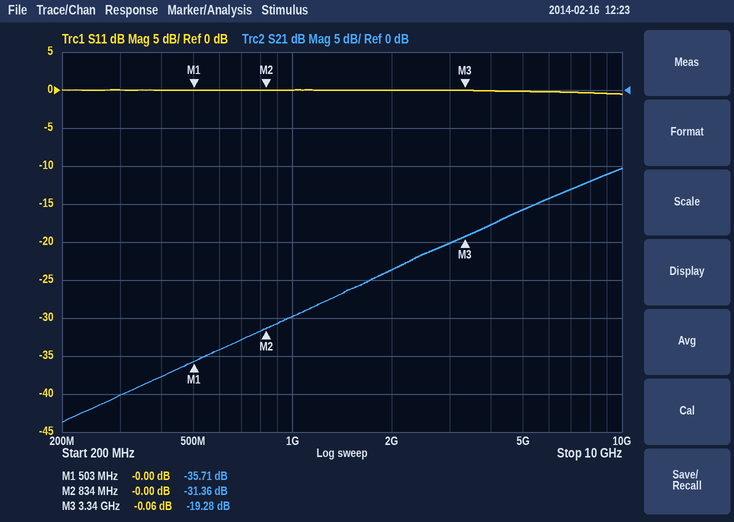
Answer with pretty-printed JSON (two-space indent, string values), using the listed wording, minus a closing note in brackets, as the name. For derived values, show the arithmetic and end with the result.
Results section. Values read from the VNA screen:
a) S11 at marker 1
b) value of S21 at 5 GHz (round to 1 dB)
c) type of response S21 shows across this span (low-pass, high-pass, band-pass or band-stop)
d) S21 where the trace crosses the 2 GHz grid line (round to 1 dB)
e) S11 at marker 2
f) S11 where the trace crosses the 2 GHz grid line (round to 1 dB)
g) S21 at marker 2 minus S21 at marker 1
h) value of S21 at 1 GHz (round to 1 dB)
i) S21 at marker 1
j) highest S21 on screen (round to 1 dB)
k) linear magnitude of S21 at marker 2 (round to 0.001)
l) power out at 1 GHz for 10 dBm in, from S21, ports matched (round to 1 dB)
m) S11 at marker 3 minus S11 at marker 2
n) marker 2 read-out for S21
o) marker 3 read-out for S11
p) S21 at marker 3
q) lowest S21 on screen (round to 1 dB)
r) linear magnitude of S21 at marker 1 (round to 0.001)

{
  "S11 at marker 1": "-0.00 dB",
  "value of S21 at 5 GHz": "-16 dB",
  "type of response S21 shows across this span": "high-pass",
  "S21 where the trace crosses the 2 GHz grid line": "-24 dB",
  "S11 at marker 2": "-0.00 dB",
  "S11 where the trace crosses the 2 GHz grid line": "0 dB",
  "S21 at marker 2 minus S21 at marker 1": "-31.36 − (-35.71) = 4.35 dB",
  "value of S21 at 1 GHz": "-30 dB",
  "S21 at marker 1": "-35.71 dB",
  "highest S21 on screen": "-10 dB",
  "linear magnitude of S21 at marker 2": "10^(-31.36/20) ≈ 0.027",
  "power out at 1 GHz for 10 dBm in, from S21, ports matched": "10 dBm + (-30 dB) = -20 dBm",
  "S11 at marker 3 minus S11 at marker 2": "-0.06 − (-0) = -0.06 dB",
  "marker 2 read-out for S21": "-31.36 dB",
  "marker 3 read-out for S11": "-0.06 dB",
  "S21 at marker 3": "-19.28 dB",
  "lowest S21 on screen": "-44 dB",
  "linear magnitude of S21 at marker 1": "10^(-35.71/20) ≈ 0.016"
}
